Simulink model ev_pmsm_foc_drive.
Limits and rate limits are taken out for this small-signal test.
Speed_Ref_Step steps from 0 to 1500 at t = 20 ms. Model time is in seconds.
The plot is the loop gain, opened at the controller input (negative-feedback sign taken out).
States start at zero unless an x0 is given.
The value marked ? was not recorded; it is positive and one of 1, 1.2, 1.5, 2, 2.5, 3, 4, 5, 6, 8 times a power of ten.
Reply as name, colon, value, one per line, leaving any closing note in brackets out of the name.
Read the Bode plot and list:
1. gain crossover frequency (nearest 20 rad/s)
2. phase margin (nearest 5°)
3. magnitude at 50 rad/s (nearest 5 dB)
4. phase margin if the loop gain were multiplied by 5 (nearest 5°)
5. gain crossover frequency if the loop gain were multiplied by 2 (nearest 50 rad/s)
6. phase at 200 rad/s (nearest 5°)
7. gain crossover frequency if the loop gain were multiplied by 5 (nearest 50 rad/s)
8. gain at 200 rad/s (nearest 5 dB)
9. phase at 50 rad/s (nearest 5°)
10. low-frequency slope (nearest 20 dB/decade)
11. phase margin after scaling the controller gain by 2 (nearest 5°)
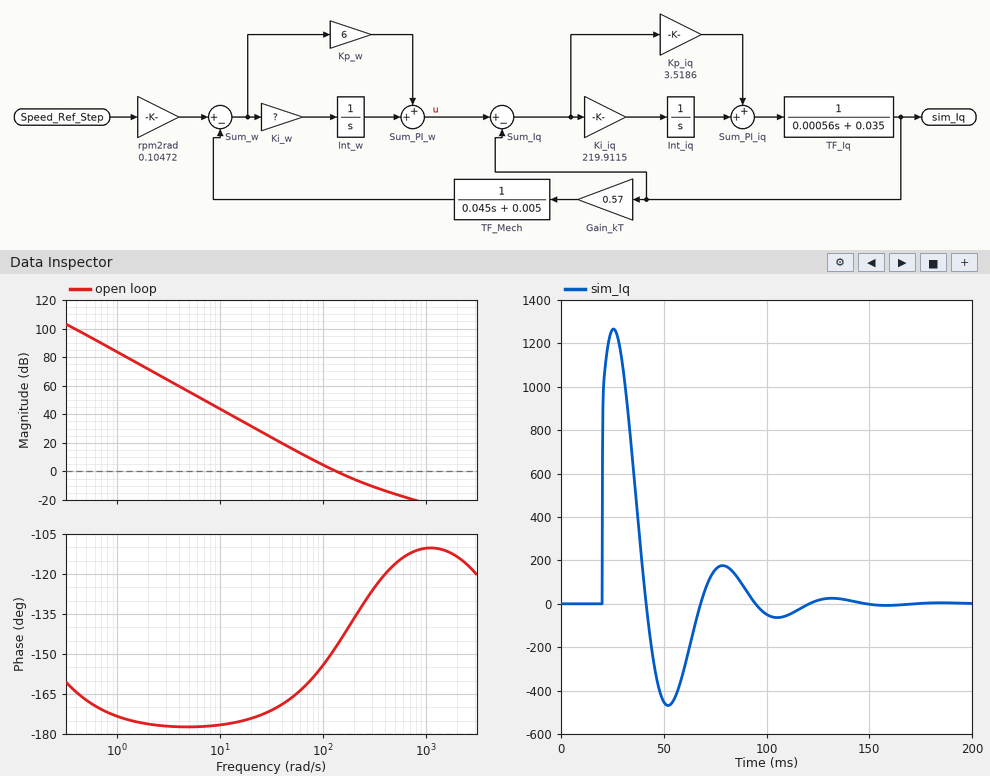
gain crossover frequency: 140 rad/s
phase margin: 35°
magnitude at 50 rad/s: 15 dB
phase margin if the loop gain were multiplied by 5: 60°
gain crossover frequency if the loop gain were multiplied by 2: 200 rad/s
phase at 200 rad/s: -135°
gain crossover frequency if the loop gain were multiplied by 5: 400 rad/s
gain at 200 rad/s: -5 dB
phase at 50 rad/s: -165°
low-frequency slope: -40 dB/decade
phase margin after scaling the controller gain by 2: 45°
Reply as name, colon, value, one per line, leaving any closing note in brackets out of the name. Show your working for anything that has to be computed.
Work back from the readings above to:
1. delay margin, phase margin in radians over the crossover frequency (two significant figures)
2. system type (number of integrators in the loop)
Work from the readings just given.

delay margin, phase margin in radians over the crossover frequency: 35 × π / 180 / 140 = 0.0044 s
system type: 2
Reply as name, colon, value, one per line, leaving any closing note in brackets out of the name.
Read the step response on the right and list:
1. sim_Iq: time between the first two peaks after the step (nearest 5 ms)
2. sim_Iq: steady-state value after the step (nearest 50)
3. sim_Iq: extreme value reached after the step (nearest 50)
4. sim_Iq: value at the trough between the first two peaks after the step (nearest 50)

sim_Iq: time between the first two peaks after the step: 55 ms
sim_Iq: steady-state value after the step: 0
sim_Iq: extreme value reached after the step: 1250
sim_Iq: value at the trough between the first two peaks after the step: -450
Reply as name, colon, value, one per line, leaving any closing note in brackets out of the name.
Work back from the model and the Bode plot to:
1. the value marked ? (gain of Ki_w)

the value marked ?: 1200
